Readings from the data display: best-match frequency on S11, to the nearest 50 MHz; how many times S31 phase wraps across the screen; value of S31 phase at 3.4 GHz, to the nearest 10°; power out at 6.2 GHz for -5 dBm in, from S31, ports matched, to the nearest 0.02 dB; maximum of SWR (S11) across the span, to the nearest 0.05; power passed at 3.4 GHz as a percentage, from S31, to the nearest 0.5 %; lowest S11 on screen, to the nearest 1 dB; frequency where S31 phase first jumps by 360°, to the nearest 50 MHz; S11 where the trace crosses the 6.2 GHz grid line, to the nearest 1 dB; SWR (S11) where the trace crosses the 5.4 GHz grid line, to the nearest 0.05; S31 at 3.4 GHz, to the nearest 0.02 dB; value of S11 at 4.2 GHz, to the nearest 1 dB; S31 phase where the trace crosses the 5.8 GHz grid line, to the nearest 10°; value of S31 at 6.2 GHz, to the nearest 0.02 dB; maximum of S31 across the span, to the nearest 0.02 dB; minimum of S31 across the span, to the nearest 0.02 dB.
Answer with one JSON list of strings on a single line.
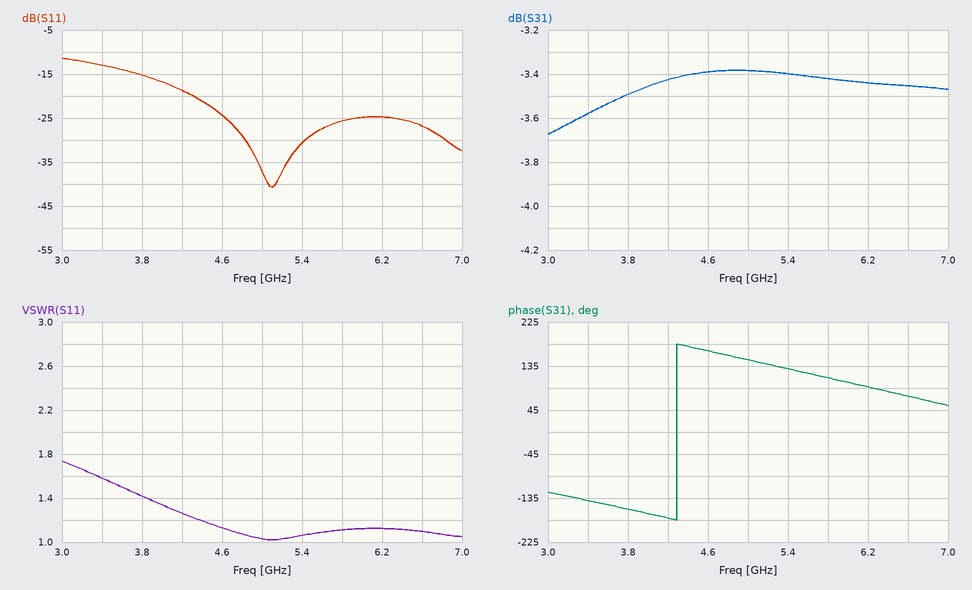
["5.10 GHz", "1", "-140°", "-8.44 dBm", "1.75", "44.0 %", "-41 dB", "4.30 GHz", "-25 dB", "1.05", "-3.58 dB", "-19 dB", "110°", "-3.44 dB", "-3.38 dB", "-3.68 dB"]
